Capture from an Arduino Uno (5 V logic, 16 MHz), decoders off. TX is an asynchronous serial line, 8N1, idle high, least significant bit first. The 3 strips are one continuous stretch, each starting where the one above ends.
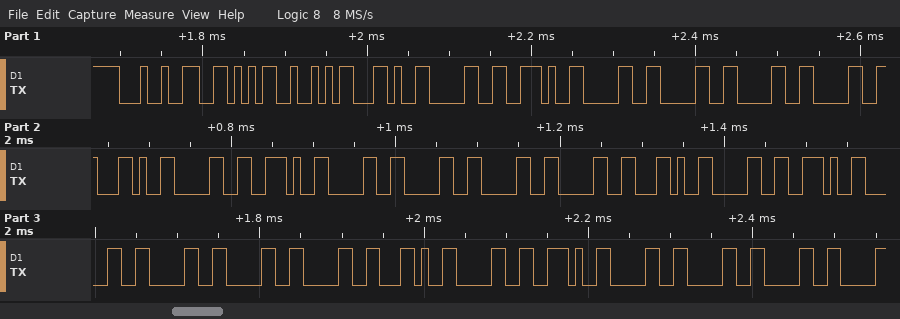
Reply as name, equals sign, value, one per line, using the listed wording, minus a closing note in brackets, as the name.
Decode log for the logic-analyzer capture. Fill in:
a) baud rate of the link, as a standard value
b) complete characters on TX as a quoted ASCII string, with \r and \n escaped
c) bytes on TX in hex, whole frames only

baud rate of the link, as a standard value = 115200 baud
complete characters on TX as a quoted ASCII string, with \r and \n escaped = "$VR,0.0000,0.0000,0.0000,0.000"
bytes on TX in hex, whole frames only = 24 56 52 2C 30 2E 30 30 30 30 2C 30 2E 30 30 30 30 2C 30 2E 30 30 30 30 2C 30 2E 30 30 30
